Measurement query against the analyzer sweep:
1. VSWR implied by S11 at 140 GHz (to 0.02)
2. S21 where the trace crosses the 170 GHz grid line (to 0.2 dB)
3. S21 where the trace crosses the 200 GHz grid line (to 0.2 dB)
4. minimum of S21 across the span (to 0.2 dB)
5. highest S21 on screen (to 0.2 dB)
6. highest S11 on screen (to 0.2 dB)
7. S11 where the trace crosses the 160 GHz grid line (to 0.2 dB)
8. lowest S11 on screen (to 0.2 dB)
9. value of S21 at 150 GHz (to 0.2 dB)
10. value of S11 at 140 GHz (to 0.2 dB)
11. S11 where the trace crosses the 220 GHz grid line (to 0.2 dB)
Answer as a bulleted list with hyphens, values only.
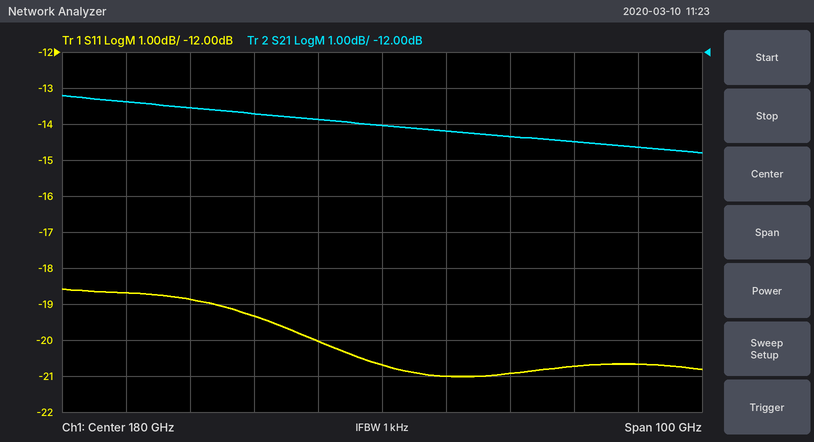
- 1.26
- -13.8 dB
- -14.4 dB
- -14.8 dB
- -13.2 dB
- -18.6 dB
- -19.4 dB
- -21.0 dB
- -13.6 dB
- -18.6 dB
- -20.6 dB
